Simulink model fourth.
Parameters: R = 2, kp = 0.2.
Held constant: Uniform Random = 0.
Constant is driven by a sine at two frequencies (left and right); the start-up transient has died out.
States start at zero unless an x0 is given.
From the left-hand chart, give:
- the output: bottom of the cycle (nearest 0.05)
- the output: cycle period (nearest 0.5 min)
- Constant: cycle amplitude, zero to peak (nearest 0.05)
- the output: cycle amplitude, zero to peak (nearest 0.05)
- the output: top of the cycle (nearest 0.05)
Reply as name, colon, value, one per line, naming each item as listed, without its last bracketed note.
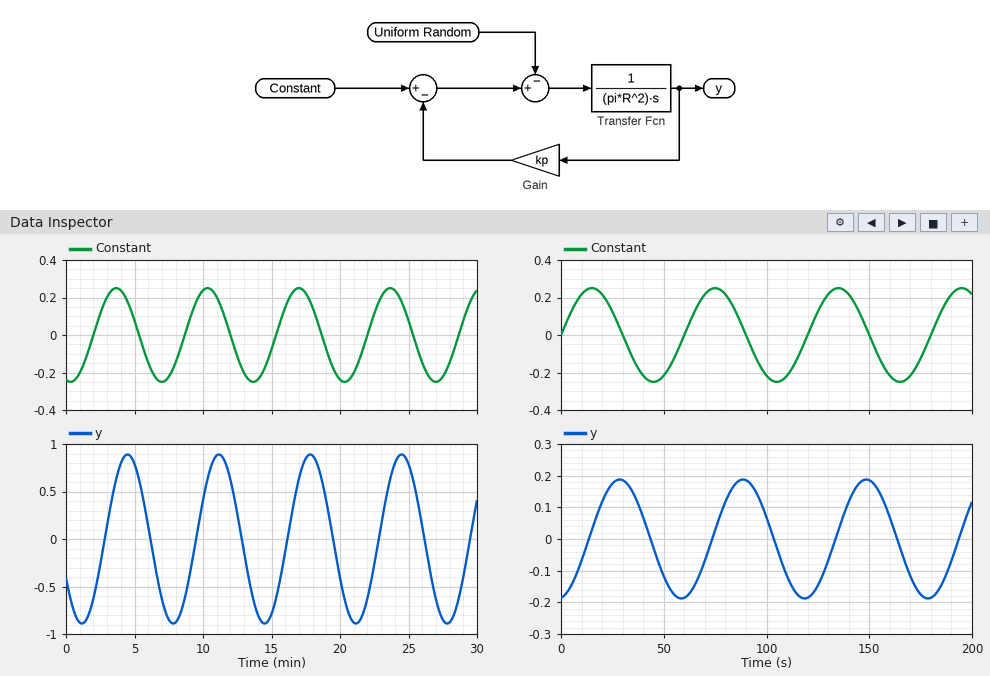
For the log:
the output: bottom of the cycle: -0.90
the output: cycle period: 6.5 min
Constant: cycle amplitude, zero to peak: 0.25
the output: cycle amplitude, zero to peak: 0.90
the output: top of the cycle: 0.90
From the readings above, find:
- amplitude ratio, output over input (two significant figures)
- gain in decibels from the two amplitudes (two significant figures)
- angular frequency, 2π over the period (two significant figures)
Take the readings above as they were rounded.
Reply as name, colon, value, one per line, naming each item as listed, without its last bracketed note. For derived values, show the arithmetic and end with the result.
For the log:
amplitude ratio, output over input: 0.9 / 0.25 = 3.6
gain in decibels from the two amplitudes: 20 log10(0.9 / 0.25) = 11 dB
angular frequency, 2π over the period: 2π / 6.5 = 0.97 rad/min
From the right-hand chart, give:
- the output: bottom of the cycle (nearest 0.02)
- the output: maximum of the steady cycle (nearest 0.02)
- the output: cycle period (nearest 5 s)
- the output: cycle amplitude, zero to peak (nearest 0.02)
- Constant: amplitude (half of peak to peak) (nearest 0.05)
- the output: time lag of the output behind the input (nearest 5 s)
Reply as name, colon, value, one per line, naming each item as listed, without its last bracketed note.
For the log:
the output: bottom of the cycle: -0.18
the output: maximum of the steady cycle: 0.18
the output: cycle period: 60 s
the output: cycle amplitude, zero to peak: 0.18
Constant: amplitude (half of peak to peak): 0.25
the output: time lag of the output behind the input: 15 s
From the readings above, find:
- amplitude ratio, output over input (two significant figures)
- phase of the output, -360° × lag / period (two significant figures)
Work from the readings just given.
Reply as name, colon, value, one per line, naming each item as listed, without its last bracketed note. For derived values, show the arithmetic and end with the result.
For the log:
amplitude ratio, output over input: 0.18 / 0.25 = 0.72
phase of the output, -360° × lag / period: -360 × 15 / 60 = -90°
